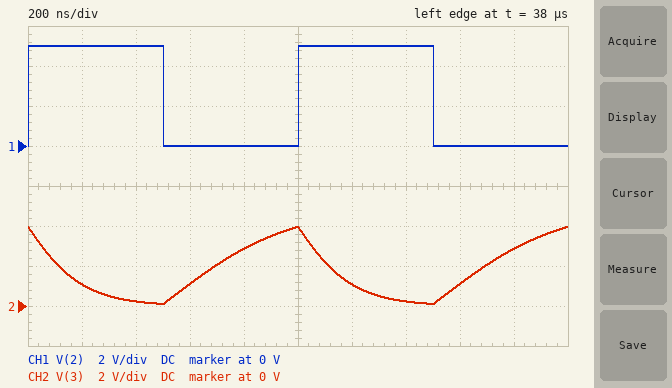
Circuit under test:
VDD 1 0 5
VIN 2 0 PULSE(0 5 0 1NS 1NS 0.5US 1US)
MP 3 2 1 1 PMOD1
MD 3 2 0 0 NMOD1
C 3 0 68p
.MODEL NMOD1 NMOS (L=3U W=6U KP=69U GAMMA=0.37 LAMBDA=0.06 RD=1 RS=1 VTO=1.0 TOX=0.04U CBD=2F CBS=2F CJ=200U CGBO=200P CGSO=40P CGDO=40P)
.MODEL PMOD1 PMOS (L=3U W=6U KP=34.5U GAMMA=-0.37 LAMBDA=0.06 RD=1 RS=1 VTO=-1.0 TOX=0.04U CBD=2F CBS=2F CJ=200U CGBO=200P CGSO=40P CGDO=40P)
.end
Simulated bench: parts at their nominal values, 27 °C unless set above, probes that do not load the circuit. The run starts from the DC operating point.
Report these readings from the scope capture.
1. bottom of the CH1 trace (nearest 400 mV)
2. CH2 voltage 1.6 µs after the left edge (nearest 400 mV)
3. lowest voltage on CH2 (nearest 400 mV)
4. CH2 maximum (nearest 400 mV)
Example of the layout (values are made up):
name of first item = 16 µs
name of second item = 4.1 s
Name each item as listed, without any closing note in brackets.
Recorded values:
bottom of the CH1 trace = 0 V
CH2 voltage 1.6 µs after the left edge = 1.2 V
lowest voltage on CH2 = 0 V
CH2 maximum = 4.0 V
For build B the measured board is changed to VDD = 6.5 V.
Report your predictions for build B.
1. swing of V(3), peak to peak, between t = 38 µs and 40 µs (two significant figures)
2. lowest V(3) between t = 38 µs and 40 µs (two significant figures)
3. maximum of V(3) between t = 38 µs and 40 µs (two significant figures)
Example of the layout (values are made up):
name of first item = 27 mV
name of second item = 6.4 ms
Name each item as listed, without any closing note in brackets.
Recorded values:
swing of V(3), peak to peak, between t = 38 µs and 40 µs = 5.7 V
lowest V(3) between t = 38 µs and 40 µs = 240 mV
maximum of V(3) between t = 38 µs and 40 µs = 5.9 V
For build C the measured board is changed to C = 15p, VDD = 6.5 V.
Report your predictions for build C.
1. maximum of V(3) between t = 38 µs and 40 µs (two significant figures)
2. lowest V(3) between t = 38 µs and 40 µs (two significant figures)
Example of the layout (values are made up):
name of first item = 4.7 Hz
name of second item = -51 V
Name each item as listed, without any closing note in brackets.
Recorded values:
maximum of V(3) between t = 38 µs and 40 µs = 6.5 V
lowest V(3) between t = 38 µs and 40 µs = 22 mV
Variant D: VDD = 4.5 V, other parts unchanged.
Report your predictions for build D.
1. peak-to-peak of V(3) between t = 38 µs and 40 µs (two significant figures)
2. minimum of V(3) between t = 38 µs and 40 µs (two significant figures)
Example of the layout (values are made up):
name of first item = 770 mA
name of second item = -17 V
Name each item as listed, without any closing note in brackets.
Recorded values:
peak-to-peak of V(3) between t = 38 µs and 40 µs = 3.2 V
minimum of V(3) between t = 38 µs and 40 µs = 75 mV
